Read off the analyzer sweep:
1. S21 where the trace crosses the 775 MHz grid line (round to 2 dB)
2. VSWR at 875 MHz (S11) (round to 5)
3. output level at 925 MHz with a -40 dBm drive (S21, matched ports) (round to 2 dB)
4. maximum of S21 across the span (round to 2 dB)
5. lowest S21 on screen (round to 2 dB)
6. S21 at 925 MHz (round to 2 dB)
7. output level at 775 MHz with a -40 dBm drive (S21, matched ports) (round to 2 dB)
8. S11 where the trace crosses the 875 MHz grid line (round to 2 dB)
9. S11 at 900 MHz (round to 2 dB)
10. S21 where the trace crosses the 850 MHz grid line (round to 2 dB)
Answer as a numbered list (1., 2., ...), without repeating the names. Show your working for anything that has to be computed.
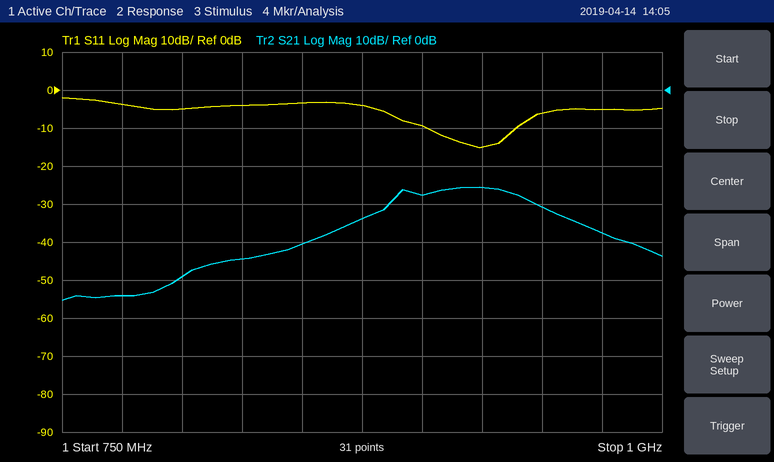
1. -54 dB
2. |Γ| = 10^(-4/20) = 0.6310; VSWR = (1 + 0.6310)/(1 − 0.6310) ≈ 4.42, so 5 to the nearest 5
3. -40 dBm + (-26 dB) = -66 dBm
4. -26 dB
5. -56 dB
6. -26 dB
7. -40 dBm + (-54 dB) = -94 dBm
8. -4 dB
9. -10 dB
10. -40 dB
